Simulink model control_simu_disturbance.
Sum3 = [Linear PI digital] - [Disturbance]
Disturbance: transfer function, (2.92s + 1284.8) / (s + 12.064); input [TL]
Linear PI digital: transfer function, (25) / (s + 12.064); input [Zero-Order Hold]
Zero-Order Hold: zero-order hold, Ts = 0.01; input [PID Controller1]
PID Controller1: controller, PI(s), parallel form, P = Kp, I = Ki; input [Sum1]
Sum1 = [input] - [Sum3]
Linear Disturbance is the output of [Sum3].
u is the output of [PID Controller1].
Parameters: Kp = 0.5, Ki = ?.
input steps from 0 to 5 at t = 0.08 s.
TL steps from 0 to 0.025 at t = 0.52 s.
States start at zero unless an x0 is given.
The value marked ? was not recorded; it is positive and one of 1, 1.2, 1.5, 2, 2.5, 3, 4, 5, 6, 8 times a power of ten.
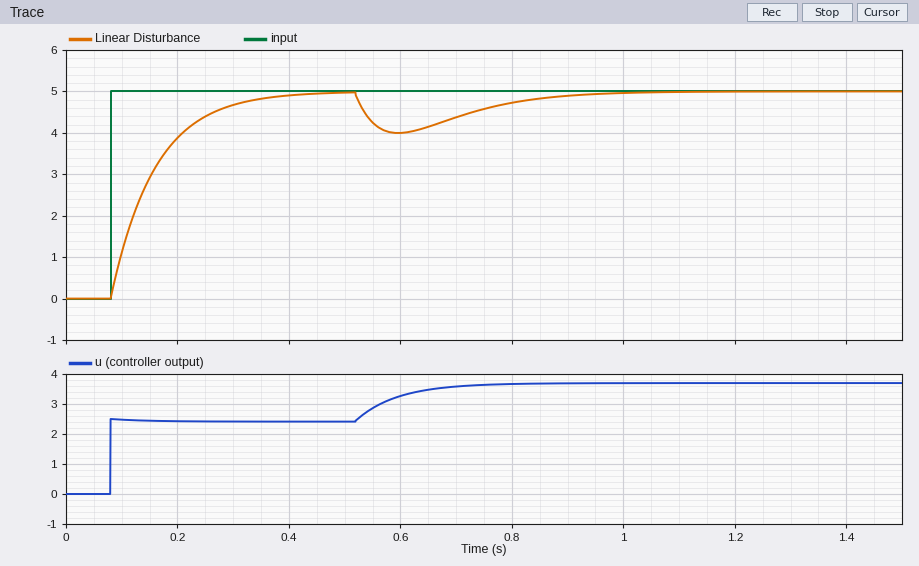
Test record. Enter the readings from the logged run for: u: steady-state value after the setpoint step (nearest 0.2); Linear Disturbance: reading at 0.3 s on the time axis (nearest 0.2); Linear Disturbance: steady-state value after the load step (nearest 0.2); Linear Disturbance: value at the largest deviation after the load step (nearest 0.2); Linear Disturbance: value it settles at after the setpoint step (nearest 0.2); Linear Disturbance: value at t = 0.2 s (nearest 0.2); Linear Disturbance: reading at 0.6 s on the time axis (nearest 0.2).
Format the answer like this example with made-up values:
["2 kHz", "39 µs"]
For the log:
["2.4", "4.6", "5.0", "4.0", "5.0", "3.8", "4.0"]
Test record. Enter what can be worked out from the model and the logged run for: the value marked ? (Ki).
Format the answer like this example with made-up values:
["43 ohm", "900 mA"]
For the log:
["6"]
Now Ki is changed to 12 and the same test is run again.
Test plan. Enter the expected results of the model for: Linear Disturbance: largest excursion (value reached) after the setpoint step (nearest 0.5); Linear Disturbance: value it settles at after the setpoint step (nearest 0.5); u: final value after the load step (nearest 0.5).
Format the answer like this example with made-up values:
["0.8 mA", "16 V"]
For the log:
["5.5", "5.0", "3.5"]
